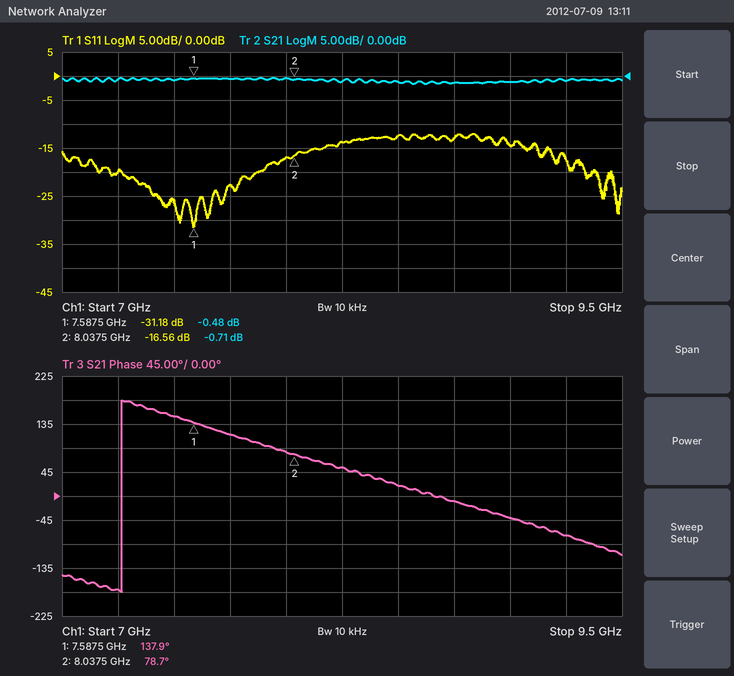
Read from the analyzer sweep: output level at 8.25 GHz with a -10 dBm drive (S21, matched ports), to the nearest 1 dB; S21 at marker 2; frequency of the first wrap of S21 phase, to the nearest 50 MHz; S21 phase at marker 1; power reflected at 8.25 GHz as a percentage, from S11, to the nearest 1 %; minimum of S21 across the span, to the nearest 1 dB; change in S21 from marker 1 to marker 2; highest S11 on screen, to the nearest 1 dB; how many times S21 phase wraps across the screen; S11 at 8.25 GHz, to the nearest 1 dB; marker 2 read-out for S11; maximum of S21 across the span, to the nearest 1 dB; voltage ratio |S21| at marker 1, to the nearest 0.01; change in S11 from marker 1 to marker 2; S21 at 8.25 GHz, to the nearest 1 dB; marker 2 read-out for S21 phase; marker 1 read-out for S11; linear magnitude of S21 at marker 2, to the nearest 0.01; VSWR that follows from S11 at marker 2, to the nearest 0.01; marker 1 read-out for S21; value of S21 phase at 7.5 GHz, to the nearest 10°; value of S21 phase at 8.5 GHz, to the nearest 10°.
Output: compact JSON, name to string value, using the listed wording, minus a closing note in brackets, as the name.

{"output level at 8.25 GHz with a -10 dBm drive (S21, matched ports), to the nearest 1 dB": "-11 dBm", "S21 at marker 2": "-0.71 dB", "frequency of the first wrap of S21 phase, to the nearest 50 MHz": "7.25 GHz", "S21 phase at marker 1": "137.9°", "power reflected at 8.25 GHz as a percentage, from S11, to the nearest 1 %": "4 %", "minimum of S21 across the span, to the nearest 1 dB": "-2 dB", "change in S21 from marker 1 to marker 2": "-0.23 dB", "highest S11 on screen, to the nearest 1 dB": "-12 dB", "how many times S21 phase wraps across the screen": "1", "S11 at 8.25 GHz, to the nearest 1 dB": "-14 dB", "marker 2 read-out for S11": "-16.56 dB", "maximum of S21 across the span, to the nearest 1 dB": "0 dB", "voltage ratio |S21| at marker 1, to the nearest 0.01": "0.95", "change in S11 from marker 1 to marker 2": "14.62 dB", "S21 at 8.25 GHz, to the nearest 1 dB": "-1 dB", "marker 2 read-out for S21 phase": "78.7°", "marker 1 read-out for S11": "-31.18 dB", "linear magnitude of S21 at marker 2, to the nearest 0.01": "0.92", "VSWR that follows from S11 at marker 2, to the nearest 0.01": "1.35", "marker 1 read-out for S21": "-0.48 dB", "value of S21 phase at 7.5 GHz, to the nearest 10°": "150°", "value of S21 phase at 8.5 GHz, to the nearest 10°": "20°"}
